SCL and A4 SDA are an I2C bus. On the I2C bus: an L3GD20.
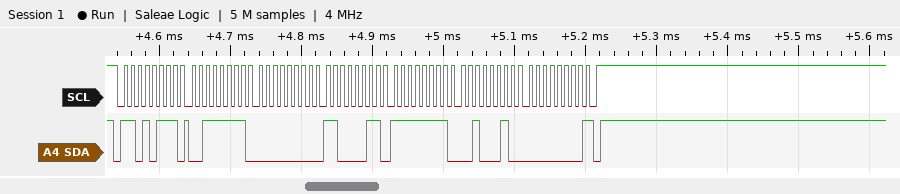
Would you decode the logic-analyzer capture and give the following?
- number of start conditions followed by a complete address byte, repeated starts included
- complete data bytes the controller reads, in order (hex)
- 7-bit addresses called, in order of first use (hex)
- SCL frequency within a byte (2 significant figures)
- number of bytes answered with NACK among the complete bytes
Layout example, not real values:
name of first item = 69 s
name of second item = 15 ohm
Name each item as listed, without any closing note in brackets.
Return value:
number of start conditions followed by a complete address byte, repeated starts included = 1
complete data bytes the controller reads, in order = 3F 00 C3 FF 22 00
7-bit addresses called, in order of first use = 0x6B
SCL frequency within a byte = 100 kHz
number of bytes answered with NACK among the complete bytes = 1
